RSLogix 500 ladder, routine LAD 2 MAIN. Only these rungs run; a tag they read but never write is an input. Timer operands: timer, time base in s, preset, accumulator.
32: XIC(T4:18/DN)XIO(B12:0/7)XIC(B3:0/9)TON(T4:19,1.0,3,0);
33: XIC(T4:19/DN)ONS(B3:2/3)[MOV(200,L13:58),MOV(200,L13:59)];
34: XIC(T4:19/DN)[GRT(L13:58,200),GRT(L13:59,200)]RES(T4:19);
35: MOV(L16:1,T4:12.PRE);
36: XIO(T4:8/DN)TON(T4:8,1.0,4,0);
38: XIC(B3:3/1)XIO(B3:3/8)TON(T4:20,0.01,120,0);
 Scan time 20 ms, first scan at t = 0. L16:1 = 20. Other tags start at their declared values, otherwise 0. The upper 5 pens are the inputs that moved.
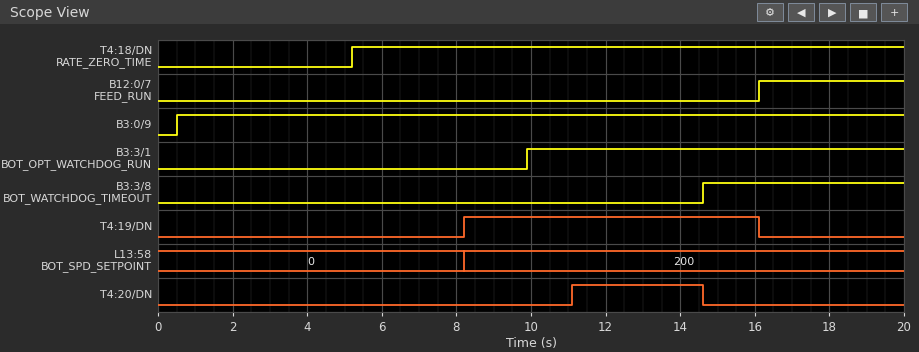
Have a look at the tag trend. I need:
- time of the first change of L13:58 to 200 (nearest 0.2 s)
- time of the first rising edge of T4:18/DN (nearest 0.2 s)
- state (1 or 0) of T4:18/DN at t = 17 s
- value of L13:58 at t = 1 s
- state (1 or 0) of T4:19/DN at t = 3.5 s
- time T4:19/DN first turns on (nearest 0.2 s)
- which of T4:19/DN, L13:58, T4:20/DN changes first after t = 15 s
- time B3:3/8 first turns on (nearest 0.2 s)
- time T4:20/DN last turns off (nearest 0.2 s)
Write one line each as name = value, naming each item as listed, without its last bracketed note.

time of the first change of L13:58 to 200 = 8.2 s
time of the first rising edge of T4:18/DN = 5.2 s
state (1 or 0) of T4:18/DN at t = 17 s = 1
value of L13:58 at t = 1 s = 0
state (1 or 0) of T4:19/DN at t = 3.5 s = 0
time T4:19/DN first turns on = 8.2 s
which of T4:19/DN, L13:58, T4:20/DN changes first after t = 15 s = T4:19/DN
time B3:3/8 first turns on = 14.6 s
time T4:20/DN last turns off = 14.6 s
